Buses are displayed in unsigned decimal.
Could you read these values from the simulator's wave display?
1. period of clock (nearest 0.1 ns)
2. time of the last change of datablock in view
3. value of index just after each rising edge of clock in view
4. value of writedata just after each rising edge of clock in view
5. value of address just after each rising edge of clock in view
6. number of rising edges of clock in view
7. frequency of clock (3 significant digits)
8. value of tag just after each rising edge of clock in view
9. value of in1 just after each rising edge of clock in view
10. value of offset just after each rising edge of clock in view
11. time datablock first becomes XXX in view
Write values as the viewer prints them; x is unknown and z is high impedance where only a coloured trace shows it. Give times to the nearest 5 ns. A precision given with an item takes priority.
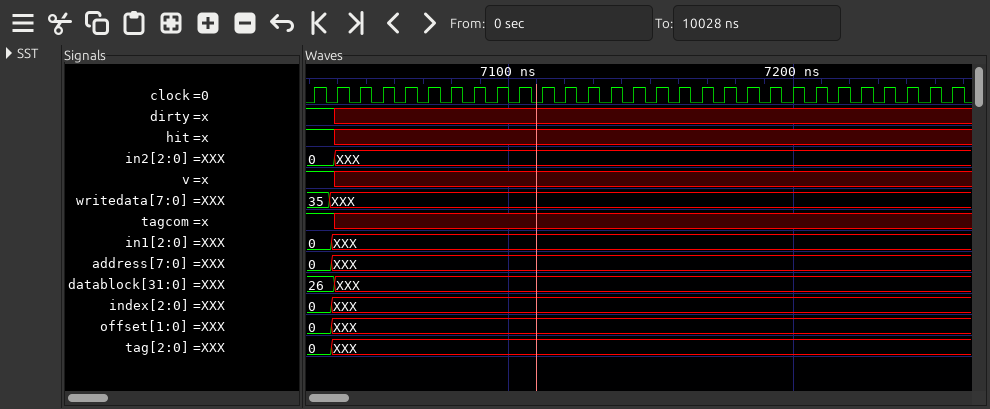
8 ns
7040 ns
0, XXX, XXX, XXX, XXX, XXX, XXX, XXX, XXX, XXX, XXX, XXX, XXX, XXX, XXX, XXX, XXX, XXX, XXX, XXX, XXX, XXX, XXX, XXX, XXX, XXX, XXX, XXX, XXX
35, XXX, XXX, XXX, XXX, XXX, XXX, XXX, XXX, XXX, XXX, XXX, XXX, XXX, XXX, XXX, XXX, XXX, XXX, XXX, XXX, XXX, XXX, XXX, XXX, XXX, XXX, XXX, XXX
0, XXX, XXX, XXX, XXX, XXX, XXX, XXX, XXX, XXX, XXX, XXX, XXX, XXX, XXX, XXX, XXX, XXX, XXX, XXX, XXX, XXX, XXX, XXX, XXX, XXX, XXX, XXX, XXX
29
125 MHz
0, XXX, XXX, XXX, XXX, XXX, XXX, XXX, XXX, XXX, XXX, XXX, XXX, XXX, XXX, XXX, XXX, XXX, XXX, XXX, XXX, XXX, XXX, XXX, XXX, XXX, XXX, XXX, XXX
0, XXX, XXX, XXX, XXX, XXX, XXX, XXX, XXX, XXX, XXX, XXX, XXX, XXX, XXX, XXX, XXX, XXX, XXX, XXX, XXX, XXX, XXX, XXX, XXX, XXX, XXX, XXX, XXX
0, XXX, XXX, XXX, XXX, XXX, XXX, XXX, XXX, XXX, XXX, XXX, XXX, XXX, XXX, XXX, XXX, XXX, XXX, XXX, XXX, XXX, XXX, XXX, XXX, XXX, XXX, XXX, XXX
7040 ns
